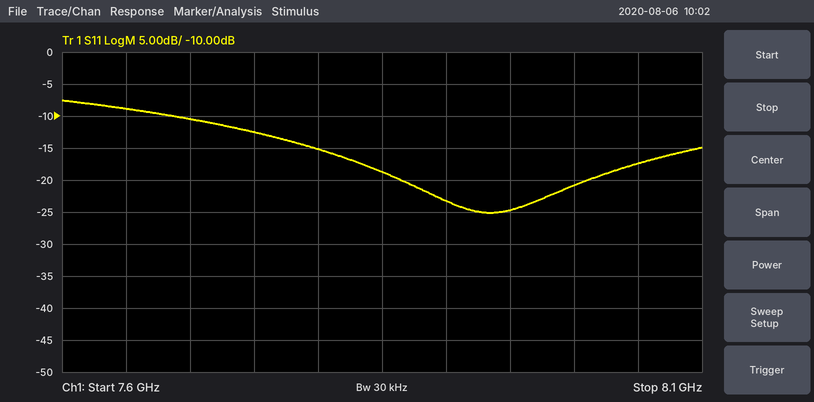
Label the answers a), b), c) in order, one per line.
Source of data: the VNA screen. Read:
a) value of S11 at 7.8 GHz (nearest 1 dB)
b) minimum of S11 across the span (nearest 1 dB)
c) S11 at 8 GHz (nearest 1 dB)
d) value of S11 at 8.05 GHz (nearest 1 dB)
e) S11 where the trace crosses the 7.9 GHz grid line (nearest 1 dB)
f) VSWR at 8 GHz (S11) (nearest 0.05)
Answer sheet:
a) -15 dB
b) -25 dB
c) -21 dB
d) -17 dB
e) -23 dB
f) 1.20
